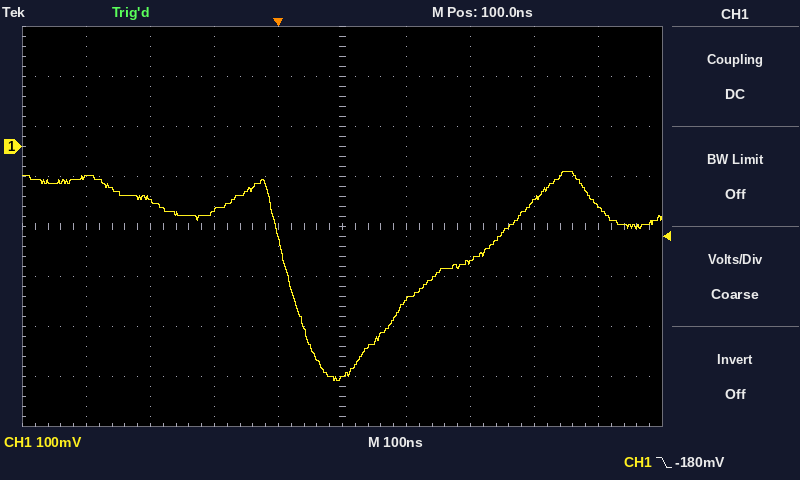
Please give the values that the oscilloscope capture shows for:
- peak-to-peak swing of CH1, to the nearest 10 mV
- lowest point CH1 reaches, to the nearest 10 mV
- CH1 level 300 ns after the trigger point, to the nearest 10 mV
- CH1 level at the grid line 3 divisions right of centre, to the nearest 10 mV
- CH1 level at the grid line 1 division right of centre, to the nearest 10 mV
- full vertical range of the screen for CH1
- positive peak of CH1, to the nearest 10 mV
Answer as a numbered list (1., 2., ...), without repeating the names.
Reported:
1. 420 mV
2. -470 mV
3. -230 mV
4. -110 mV
5. -310 mV
6. 800 mV
7. -50 mV
